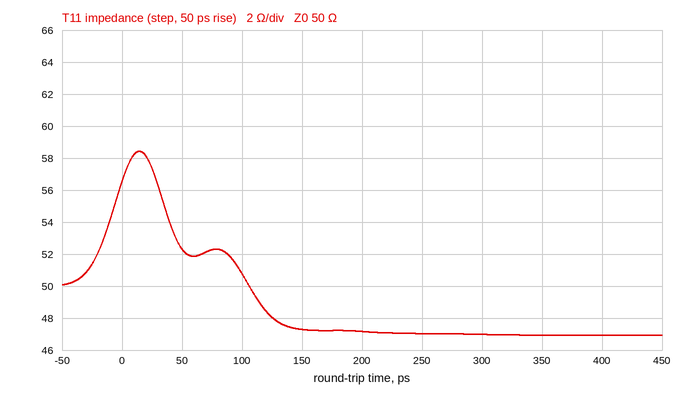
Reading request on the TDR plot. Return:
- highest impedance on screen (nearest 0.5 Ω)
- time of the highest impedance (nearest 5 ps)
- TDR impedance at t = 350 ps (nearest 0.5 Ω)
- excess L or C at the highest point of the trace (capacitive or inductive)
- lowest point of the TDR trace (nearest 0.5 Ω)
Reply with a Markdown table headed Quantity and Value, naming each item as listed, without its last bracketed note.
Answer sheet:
| Quantity | Value |
|---|---|
| highest impedance on screen | 58.5 Ω |
| time of the highest impedance | 15 ps |
| TDR impedance at t = 350 ps | 47.0 Ω |
| excess L or C at the highest point of the trace | inductive |
| lowest point of the TDR trace | 47.0 Ω |
